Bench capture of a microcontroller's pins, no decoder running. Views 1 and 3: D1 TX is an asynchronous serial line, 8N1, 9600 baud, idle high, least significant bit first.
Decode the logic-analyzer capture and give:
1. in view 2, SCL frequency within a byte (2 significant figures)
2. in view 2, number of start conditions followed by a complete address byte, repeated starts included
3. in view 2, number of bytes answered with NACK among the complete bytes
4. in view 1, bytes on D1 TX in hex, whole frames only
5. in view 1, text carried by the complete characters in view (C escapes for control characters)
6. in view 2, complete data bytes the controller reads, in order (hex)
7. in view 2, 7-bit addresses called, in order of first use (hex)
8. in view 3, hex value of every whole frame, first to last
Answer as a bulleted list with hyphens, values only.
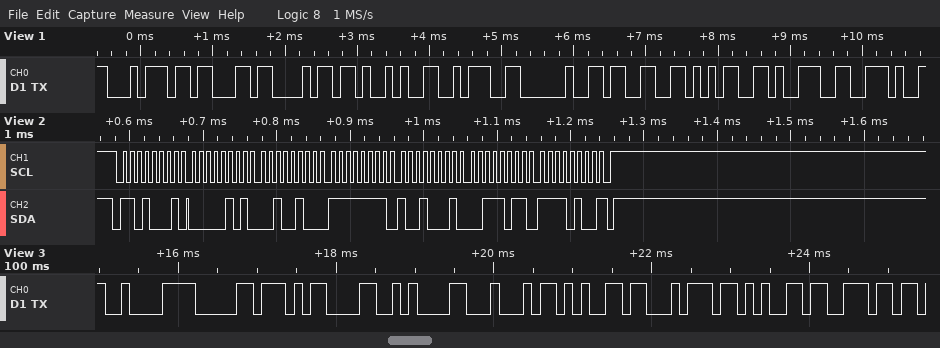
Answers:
- 100 kHz
- 1
- 1
- 74 63 68 29 3A 20 33 35 39 2E
- "tch): 359."
- 05 24 FF 91 3B F4
- 0x68
- C2 B0 0D 0A 44 65 74 65 6E
